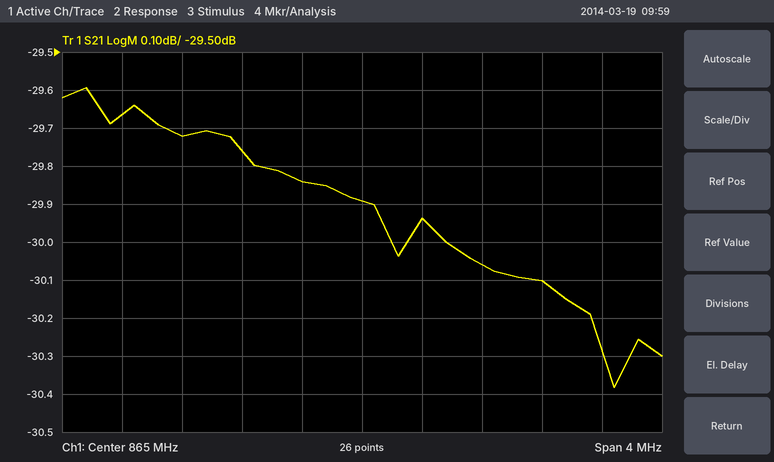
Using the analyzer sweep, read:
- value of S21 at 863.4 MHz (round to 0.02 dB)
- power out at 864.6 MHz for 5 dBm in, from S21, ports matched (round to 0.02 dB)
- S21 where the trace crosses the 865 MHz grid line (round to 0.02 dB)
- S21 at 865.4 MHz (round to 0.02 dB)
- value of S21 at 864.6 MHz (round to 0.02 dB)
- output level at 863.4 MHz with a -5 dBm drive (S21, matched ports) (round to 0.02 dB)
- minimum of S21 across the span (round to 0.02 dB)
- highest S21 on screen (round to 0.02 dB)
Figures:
-29.66 dB
-24.84 dBm
-29.90 dB
-29.94 dB
-29.84 dB
-34.66 dBm
-30.38 dB
-29.60 dB
